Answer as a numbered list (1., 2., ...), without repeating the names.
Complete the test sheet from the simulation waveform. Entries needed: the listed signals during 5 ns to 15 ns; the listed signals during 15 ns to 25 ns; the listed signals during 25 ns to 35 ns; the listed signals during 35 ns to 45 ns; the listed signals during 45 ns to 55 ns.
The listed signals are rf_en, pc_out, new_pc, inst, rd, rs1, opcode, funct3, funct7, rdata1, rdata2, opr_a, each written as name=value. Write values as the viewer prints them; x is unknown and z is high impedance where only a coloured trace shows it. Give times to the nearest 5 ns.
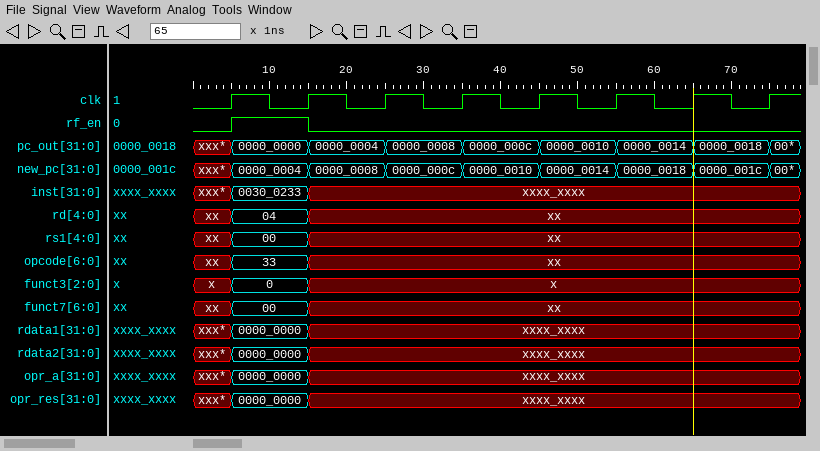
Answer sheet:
1. rf_en=1, pc_out=0000_0000, new_pc=0000_0004, inst=0030_0233, rd=04, rs1=00, opcode=33, funct3=0, funct7=00, rdata1=0000_0000, rdata2=0000_0000, opr_a=0000_0000
2. rf_en=0, pc_out=0000_0004, new_pc=0000_0008, inst=xxxx_xxxx, rd=xx, rs1=xx, opcode=xx, funct3=x, funct7=xx, rdata1=xxxx_xxxx, rdata2=xxxx_xxxx, opr_a=xxxx_xxxx
3. rf_en=0, pc_out=0000_0008, new_pc=0000_000c, inst=xxxx_xxxx, rd=xx, rs1=xx, opcode=xx, funct3=x, funct7=xx, rdata1=xxxx_xxxx, rdata2=xxxx_xxxx, opr_a=xxxx_xxxx
4. rf_en=0, pc_out=0000_000c, new_pc=0000_0010, inst=xxxx_xxxx, rd=xx, rs1=xx, opcode=xx, funct3=x, funct7=xx, rdata1=xxxx_xxxx, rdata2=xxxx_xxxx, opr_a=xxxx_xxxx
5. rf_en=0, pc_out=0000_0010, new_pc=0000_0014, inst=xxxx_xxxx, rd=xx, rs1=xx, opcode=xx, funct3=x, funct7=xx, rdata1=xxxx_xxxx, rdata2=xxxx_xxxx, opr_a=xxxx_xxxx
